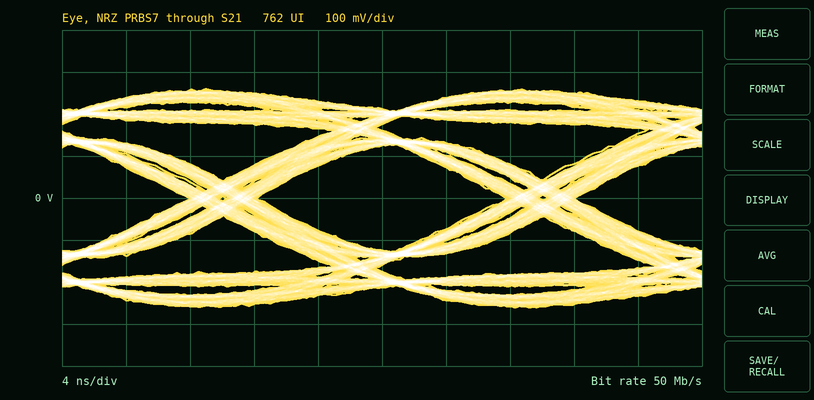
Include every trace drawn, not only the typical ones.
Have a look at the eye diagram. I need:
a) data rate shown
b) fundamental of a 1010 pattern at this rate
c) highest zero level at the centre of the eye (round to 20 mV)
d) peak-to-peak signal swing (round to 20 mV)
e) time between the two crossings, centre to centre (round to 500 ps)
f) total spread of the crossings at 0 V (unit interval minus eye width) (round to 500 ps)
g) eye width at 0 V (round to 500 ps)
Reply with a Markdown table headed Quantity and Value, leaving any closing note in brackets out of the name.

| Quantity | Value |
|---|---|
| data rate shown | 50 Mb/s |
| fundamental of a 1010 pattern at this rate | 25 MHz |
| highest zero level at the centre of the eye | -120 mV |
| peak-to-peak signal swing | 520 mV |
| time between the two crossings, centre to centre | 20.0 ns |
| total spread of the crossings at 0 V (unit interval minus eye width) | 4.5 ns |
| eye width at 0 V | 15.5 ns |
